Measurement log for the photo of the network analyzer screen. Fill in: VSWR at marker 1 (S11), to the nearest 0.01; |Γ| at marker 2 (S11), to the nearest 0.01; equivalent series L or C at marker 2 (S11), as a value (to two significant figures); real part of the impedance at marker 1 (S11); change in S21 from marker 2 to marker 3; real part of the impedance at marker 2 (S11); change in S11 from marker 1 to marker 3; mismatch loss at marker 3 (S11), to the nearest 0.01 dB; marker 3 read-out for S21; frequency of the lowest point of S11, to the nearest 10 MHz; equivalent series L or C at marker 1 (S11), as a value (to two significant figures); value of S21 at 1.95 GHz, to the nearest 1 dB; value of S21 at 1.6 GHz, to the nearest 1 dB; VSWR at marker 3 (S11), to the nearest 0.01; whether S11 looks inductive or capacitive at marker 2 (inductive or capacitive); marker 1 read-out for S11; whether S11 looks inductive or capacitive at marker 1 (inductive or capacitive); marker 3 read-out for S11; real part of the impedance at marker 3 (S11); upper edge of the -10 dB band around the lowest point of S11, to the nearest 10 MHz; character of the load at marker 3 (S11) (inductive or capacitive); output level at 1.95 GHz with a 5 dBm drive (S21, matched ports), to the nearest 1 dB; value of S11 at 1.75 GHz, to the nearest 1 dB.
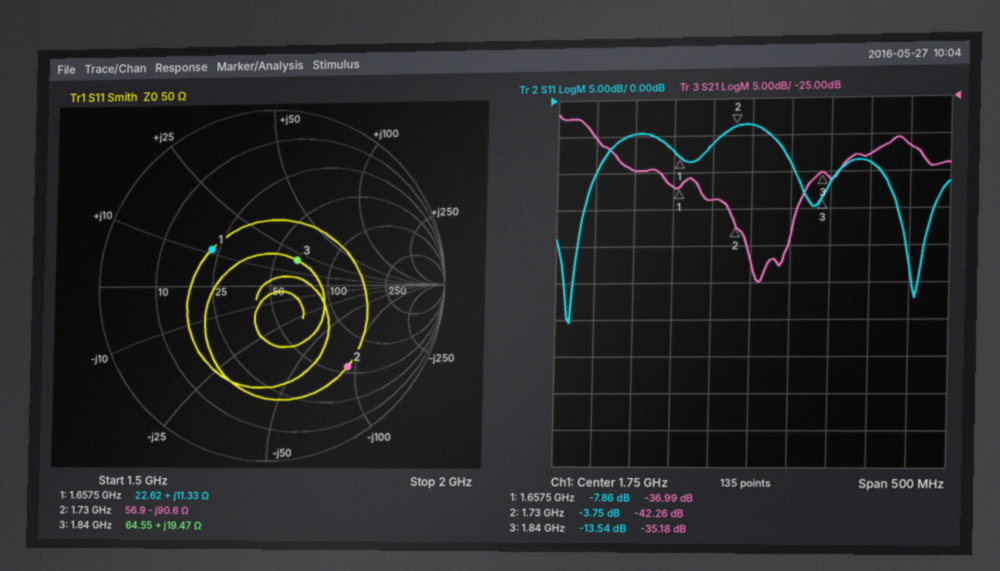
2.36
0.65
1.0 pF
22.62 Ω
7.08 dB
56.9 Ω
-5.68 dB
0.20 dB
-35.18 dB
1.52 GHz
1.1 nH
-32 dB
-35 dB
1.53
capacitive
-7.86 dB
inductive
-13.54 dB
64.55 Ω
1.55 GHz
inductive
-27 dBm
-4 dB
